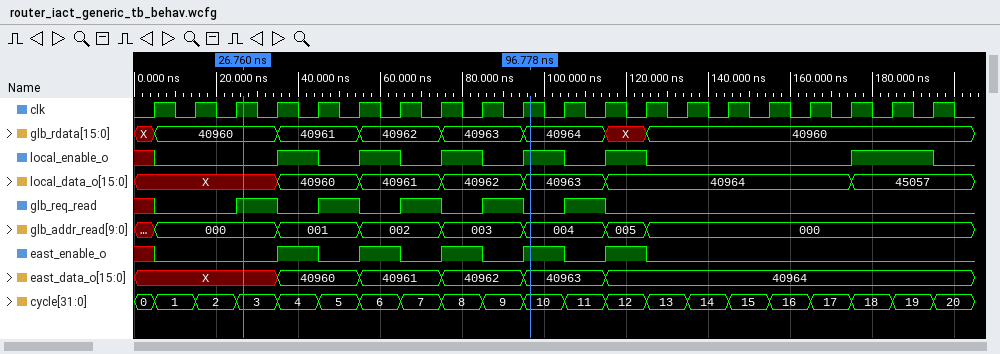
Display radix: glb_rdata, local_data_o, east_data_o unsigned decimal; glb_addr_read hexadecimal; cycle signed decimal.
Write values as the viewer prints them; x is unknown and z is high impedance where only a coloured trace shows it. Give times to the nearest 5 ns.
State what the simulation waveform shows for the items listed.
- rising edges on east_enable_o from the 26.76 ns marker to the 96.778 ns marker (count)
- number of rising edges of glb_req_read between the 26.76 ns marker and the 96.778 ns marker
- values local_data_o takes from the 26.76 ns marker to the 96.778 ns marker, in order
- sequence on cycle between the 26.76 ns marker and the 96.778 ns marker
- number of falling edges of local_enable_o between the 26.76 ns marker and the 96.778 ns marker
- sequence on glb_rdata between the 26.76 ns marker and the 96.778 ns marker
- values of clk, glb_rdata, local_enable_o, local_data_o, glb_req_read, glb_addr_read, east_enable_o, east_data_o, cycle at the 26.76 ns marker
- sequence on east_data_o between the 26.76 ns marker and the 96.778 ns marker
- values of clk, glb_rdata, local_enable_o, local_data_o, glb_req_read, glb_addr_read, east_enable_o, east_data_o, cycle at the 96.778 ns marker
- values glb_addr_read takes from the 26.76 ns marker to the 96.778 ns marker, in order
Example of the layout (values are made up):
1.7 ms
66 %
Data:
4
3
X, 40960, 40961, 40962, 40963
3, 4, 5, 6, 7, 8, 9, 10
3
40960, 40961, 40962, 40963, 40964
clk=1, glb_rdata=40960, local_enable_o=0, local_data_o=X, glb_req_read=1, glb_addr_read=000, east_enable_o=0, east_data_o=X, cycle=3
X, 40960, 40961, 40962, 40963
clk=1, glb_rdata=40964, local_enable_o=1, local_data_o=40963, glb_req_read=0, glb_addr_read=004, east_enable_o=1, east_data_o=40963, cycle=10
000, 001, 002, 003, 004
